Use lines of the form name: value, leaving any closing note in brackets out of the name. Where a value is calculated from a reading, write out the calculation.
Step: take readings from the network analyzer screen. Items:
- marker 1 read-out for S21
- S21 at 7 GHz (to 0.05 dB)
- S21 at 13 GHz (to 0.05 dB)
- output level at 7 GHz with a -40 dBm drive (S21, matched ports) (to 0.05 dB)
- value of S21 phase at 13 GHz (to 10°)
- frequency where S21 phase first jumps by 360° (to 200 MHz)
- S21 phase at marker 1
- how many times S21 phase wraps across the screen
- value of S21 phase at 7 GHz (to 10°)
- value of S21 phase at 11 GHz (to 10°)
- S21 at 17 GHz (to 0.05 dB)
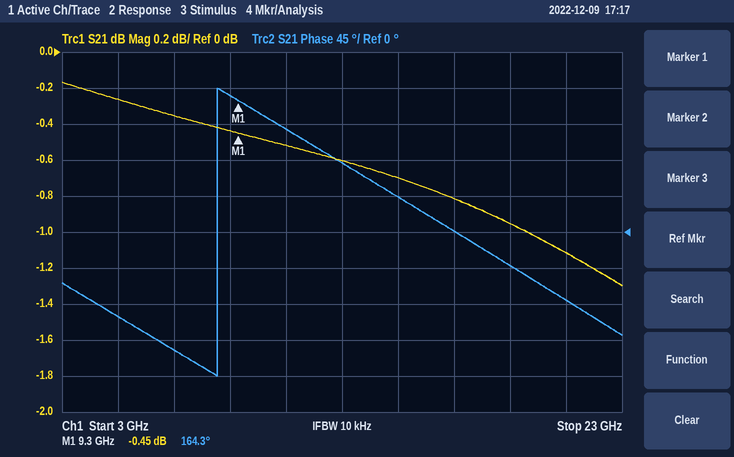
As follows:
marker 1 read-out for S21: -0.45 dB
S21 at 7 GHz: -0.35 dB
S21 at 13 GHz: -0.60 dB
output level at 7 GHz with a -40 dBm drive (S21, matched ports): -40 dBm + (-0.35 dB) = -40.35 dBm
value of S21 phase at 13 GHz: 90°
frequency where S21 phase first jumps by 360°: 8.6 GHz
S21 phase at marker 1: 164.3°
how many times S21 phase wraps across the screen: 1
value of S21 phase at 7 GHz: -150°
value of S21 phase at 11 GHz: 130°
S21 at 17 GHz: -0.80 dB
